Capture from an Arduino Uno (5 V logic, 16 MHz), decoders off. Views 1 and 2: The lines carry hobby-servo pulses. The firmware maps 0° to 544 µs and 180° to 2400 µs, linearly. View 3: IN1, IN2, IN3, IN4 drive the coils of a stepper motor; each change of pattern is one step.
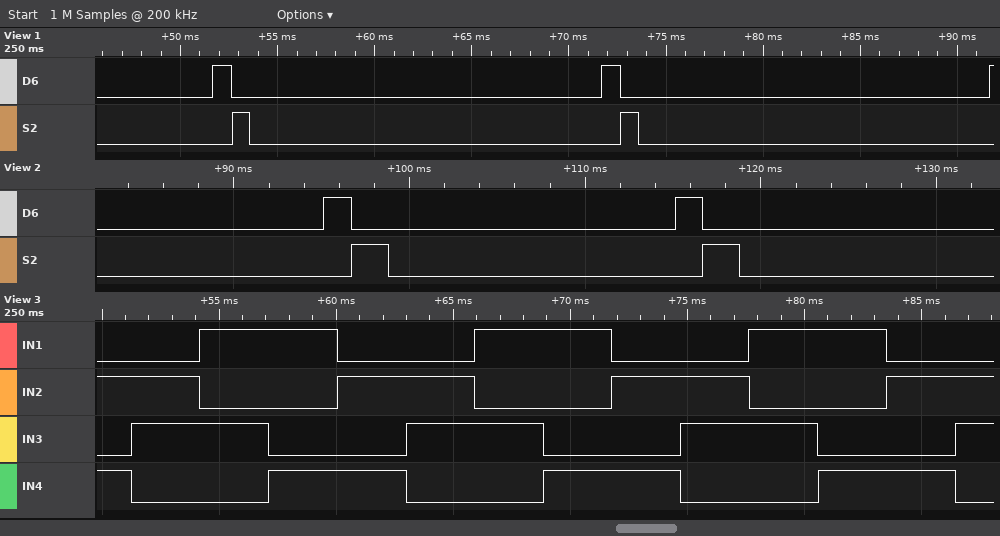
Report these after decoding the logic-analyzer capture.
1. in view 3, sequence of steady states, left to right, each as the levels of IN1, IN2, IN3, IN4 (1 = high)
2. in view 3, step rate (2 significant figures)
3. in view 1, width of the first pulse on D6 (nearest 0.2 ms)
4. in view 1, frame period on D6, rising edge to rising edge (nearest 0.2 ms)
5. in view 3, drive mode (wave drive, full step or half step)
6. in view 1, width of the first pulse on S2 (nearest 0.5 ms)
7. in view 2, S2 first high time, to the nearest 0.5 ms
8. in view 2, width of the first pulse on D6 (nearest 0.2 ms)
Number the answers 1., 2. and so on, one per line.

1. 0101 0110 1010 1001 0101 0110 1010 1001 0101 0110 1010 1001 0101 0110
2. 340 steps/s
3. 1.0 ms
4. 20.0 ms
5. full step
6. 1.0 ms
7. 2.0 ms
8. 1.6 ms
